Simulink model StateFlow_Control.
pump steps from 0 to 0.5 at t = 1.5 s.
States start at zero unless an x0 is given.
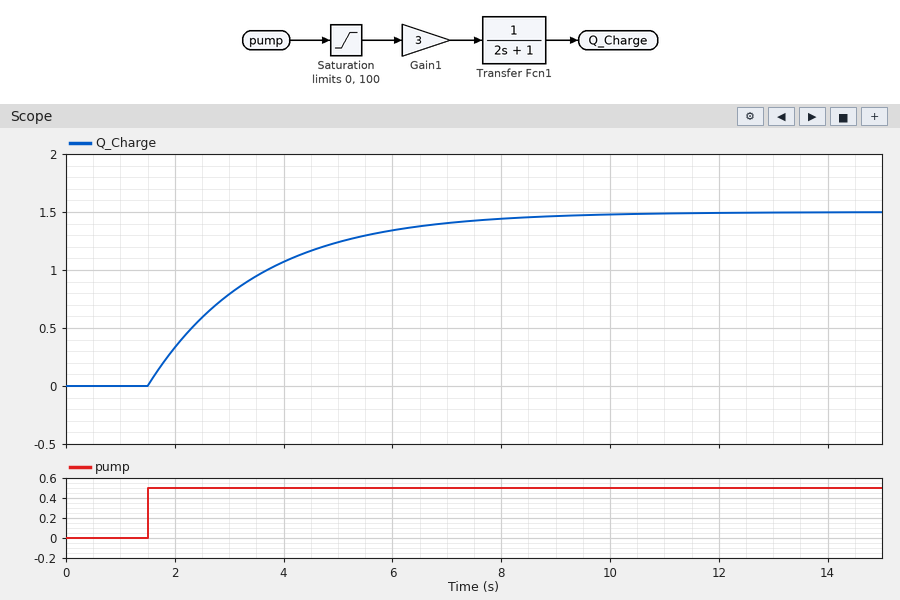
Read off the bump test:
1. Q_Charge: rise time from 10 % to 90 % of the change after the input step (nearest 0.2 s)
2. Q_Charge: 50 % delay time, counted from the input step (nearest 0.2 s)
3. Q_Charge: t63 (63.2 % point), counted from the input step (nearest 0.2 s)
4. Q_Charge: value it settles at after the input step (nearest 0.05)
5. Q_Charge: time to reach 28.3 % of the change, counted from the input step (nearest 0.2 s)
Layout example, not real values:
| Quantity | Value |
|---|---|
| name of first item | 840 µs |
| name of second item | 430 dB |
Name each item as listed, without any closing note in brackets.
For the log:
| Quantity | Value |
|---|---|
| Q_Charge: rise time from 10 % to 90 % of the change after the input step | 4.4 s |
| Q_Charge: 50 % delay time, counted from the input step | 1.4 s |
| Q_Charge: t63 (63.2 % point), counted from the input step | 2.0 s |
| Q_Charge: value it settles at after the input step | 1.50 |
| Q_Charge: time to reach 28.3 % of the change, counted from the input step | 0.6 s |
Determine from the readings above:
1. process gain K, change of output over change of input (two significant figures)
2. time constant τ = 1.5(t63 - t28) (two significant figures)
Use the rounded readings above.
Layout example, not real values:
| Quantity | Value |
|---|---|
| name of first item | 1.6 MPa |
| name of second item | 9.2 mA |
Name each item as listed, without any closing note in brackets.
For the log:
| Quantity | Value |
|---|---|
| process gain K, change of output over change of input | 3.0 |
| time constant τ = 1.5(t63 - t28) | 2.1 s |
